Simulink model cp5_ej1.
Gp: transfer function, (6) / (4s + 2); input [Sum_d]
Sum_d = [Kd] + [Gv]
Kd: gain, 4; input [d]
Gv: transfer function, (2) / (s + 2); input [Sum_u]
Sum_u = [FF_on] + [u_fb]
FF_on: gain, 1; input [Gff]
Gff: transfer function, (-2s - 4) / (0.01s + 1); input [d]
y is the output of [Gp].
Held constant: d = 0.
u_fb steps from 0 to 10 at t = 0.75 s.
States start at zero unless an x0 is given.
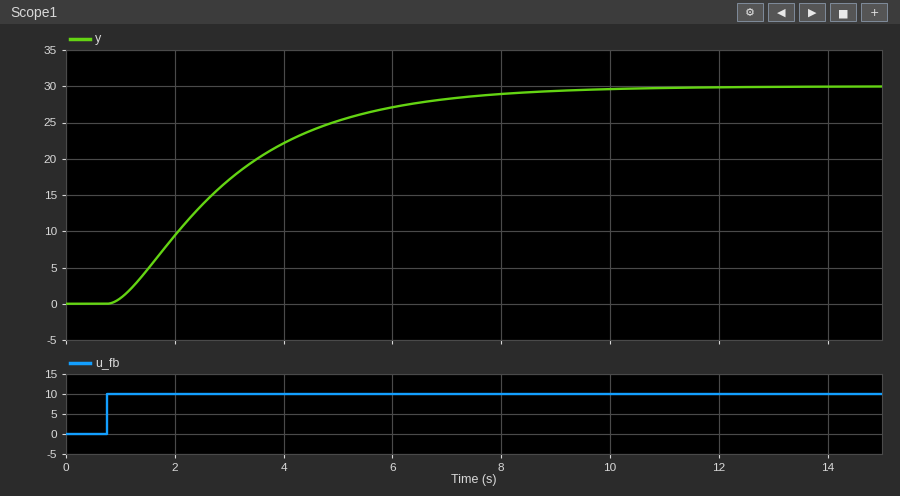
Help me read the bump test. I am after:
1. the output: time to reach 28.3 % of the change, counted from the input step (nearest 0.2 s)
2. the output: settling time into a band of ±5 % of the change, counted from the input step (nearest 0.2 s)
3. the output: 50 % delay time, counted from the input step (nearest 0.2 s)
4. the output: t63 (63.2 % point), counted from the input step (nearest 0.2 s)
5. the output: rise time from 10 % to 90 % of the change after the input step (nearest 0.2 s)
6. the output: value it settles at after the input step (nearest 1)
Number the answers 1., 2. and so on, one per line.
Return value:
1. 1.2 s
2. 6.6 s
3. 2.0 s
4. 2.6 s
5. 4.6 s
6. 30
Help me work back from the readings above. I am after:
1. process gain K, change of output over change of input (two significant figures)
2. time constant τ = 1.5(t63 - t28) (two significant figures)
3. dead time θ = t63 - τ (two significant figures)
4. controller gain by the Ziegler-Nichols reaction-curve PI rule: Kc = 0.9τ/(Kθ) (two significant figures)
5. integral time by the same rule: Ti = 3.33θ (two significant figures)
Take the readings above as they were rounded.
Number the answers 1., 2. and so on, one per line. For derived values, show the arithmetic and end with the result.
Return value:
1. (30 - 0) / 10 = 3.0
2. 1.5 × (2.6 - 1.2) = 2.1 s
3. 2.6 - 2.1 = 0.50 s
4. 0.9 × 2.1 / (3 × 0.5) = 1.3
5. 3.33 × 0.5 = 1.7 s
